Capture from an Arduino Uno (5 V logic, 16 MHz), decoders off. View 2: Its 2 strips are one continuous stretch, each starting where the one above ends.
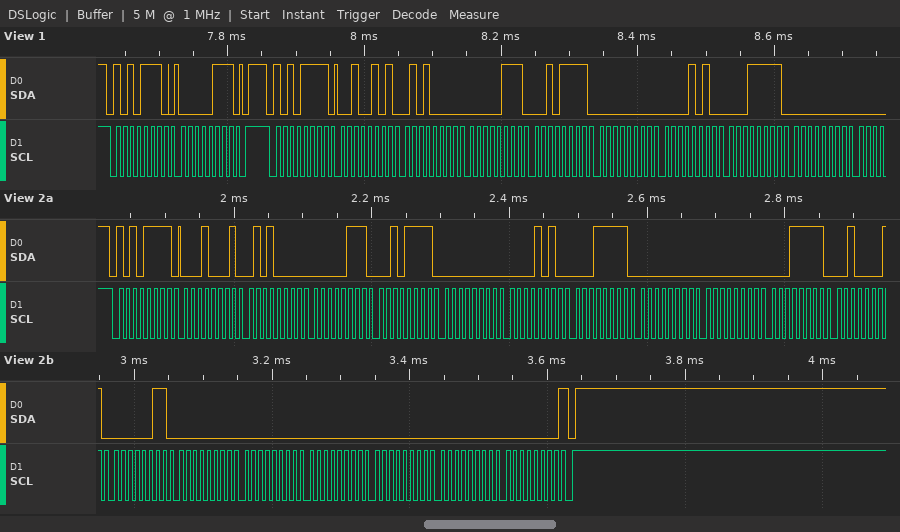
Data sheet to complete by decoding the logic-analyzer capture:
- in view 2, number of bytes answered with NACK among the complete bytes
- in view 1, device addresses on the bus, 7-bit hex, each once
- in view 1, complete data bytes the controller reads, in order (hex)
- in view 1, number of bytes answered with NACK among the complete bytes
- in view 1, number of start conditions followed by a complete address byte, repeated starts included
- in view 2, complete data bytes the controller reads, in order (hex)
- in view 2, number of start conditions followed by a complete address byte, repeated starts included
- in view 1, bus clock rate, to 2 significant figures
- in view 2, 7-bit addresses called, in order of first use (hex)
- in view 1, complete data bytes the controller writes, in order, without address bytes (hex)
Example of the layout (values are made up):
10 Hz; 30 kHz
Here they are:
1; 0x57; 25 50 07 2F 00 0A 1F 00; 0; 2; 11 50 07 2F 00 0A 1F 00 00 1F 21 03 00 00 00 00 00 00; 1; 100 kHz; 0x57; 07
